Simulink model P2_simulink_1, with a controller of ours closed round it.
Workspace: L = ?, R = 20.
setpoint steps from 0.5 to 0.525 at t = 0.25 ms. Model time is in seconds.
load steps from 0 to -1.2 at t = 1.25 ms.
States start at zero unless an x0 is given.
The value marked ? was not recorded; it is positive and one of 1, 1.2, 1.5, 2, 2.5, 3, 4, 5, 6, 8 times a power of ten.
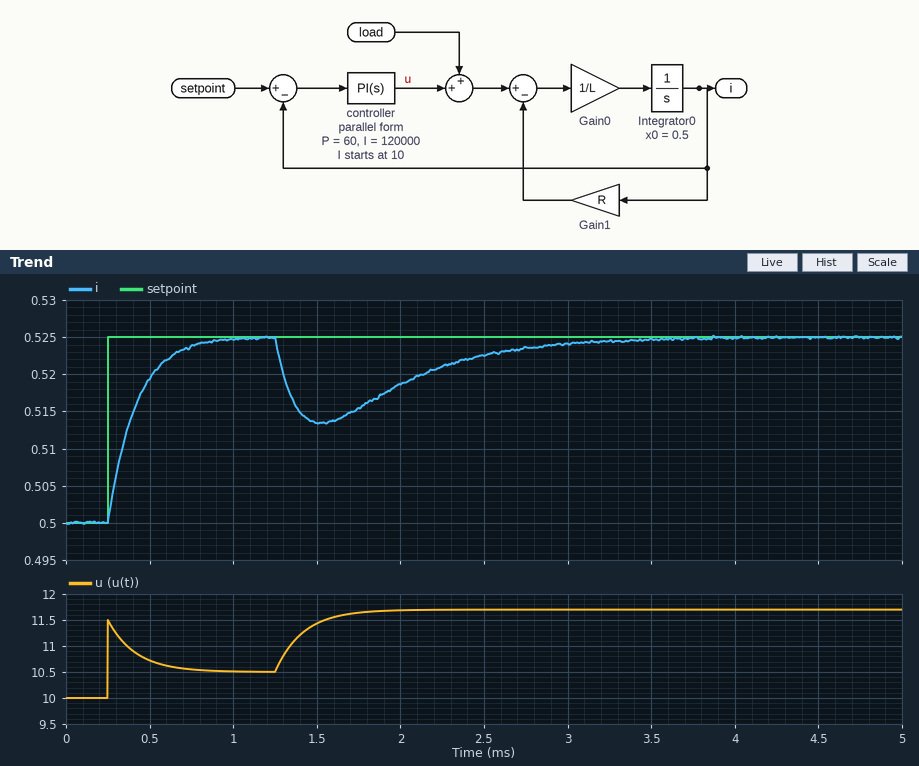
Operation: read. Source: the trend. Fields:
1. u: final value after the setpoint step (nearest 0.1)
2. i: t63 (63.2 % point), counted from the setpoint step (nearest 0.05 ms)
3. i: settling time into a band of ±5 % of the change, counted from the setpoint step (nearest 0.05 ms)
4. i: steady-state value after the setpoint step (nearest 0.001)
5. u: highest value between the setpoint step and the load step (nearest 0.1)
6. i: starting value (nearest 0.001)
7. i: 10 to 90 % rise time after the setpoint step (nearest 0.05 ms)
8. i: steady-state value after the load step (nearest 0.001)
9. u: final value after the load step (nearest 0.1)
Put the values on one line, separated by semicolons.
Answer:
10.5; 0.15 ms; 0.50 ms; 0.525; 11.5; 0.500; 0.35 ms; 0.525; 11.7
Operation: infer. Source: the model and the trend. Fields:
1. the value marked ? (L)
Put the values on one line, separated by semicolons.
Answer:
0.01
